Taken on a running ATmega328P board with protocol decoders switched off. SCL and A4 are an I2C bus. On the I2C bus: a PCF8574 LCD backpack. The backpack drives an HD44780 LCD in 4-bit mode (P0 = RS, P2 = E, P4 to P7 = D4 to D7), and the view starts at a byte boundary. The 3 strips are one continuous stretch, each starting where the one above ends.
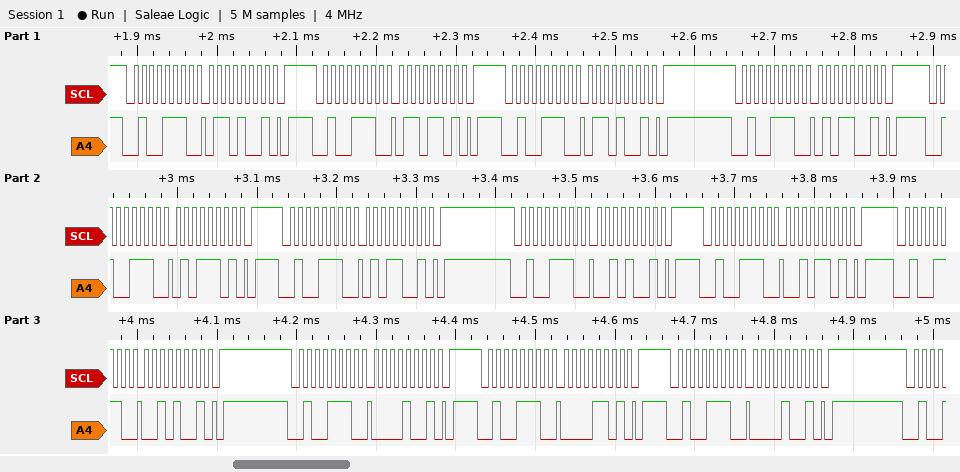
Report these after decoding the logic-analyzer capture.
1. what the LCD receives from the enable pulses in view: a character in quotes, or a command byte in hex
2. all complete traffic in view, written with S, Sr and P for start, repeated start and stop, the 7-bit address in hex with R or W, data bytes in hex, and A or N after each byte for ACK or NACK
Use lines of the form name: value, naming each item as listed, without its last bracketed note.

what the LCD receives from the enable pulses in view: a character in quotes, or a command byte in hex: 'e' ' '
all complete traffic in view, written with S, Sr and P for start, repeated start and stop, the 7-bit address in hex with R or W, data bytes in hex, and A or N after each byte for ACK or NACK: S 27W A 69 A P S 27W A 6D A P S 27W A 69 A P S 27W A 59 A P S 27W A 5D A P S 27W A 59 A P S 27W A 29 A P S 27W A 2D A P S 27W A 29 A P S 27W A 09 A P S 27W A 0D A P S 27W A 09 A P
